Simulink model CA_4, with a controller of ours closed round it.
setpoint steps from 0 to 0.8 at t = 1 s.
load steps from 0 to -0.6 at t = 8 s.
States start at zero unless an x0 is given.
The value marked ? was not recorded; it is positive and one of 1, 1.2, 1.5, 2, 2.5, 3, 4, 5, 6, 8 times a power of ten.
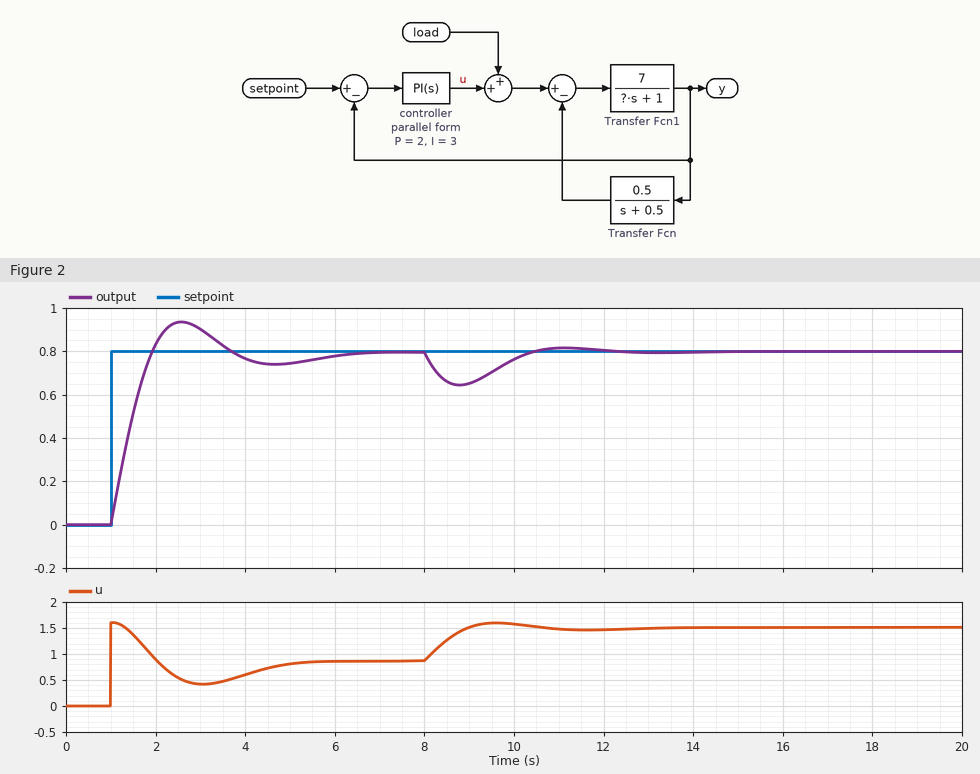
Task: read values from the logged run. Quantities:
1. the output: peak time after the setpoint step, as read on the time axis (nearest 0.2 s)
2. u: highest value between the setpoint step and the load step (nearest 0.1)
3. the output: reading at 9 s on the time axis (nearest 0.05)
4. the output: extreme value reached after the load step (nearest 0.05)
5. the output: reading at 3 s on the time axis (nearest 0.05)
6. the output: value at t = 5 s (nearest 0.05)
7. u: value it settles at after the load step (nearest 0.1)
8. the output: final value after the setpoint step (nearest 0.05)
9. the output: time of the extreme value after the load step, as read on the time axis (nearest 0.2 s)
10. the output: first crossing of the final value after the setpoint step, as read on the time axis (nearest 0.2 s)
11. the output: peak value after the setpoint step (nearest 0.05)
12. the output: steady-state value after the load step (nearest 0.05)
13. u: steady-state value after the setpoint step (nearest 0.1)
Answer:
2.6 s
1.6
0.65
0.65
0.90
0.75
1.5
0.80
8.8 s
2.0 s
0.95
0.80
0.9
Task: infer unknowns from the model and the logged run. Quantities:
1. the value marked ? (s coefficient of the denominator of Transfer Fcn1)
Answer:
10
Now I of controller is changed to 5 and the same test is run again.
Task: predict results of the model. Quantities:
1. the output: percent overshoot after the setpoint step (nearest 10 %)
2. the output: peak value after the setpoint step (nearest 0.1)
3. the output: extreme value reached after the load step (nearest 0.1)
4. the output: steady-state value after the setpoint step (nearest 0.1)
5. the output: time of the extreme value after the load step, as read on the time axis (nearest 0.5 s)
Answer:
30 %
1.0
0.7
0.8
8.5 s
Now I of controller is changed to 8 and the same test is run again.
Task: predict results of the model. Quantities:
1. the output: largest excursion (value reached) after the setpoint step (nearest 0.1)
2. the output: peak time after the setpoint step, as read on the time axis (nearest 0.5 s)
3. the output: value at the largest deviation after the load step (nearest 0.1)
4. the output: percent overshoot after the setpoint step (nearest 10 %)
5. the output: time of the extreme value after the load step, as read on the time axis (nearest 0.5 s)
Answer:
1.1
2.0 s
0.7
40 %
8.5 s
